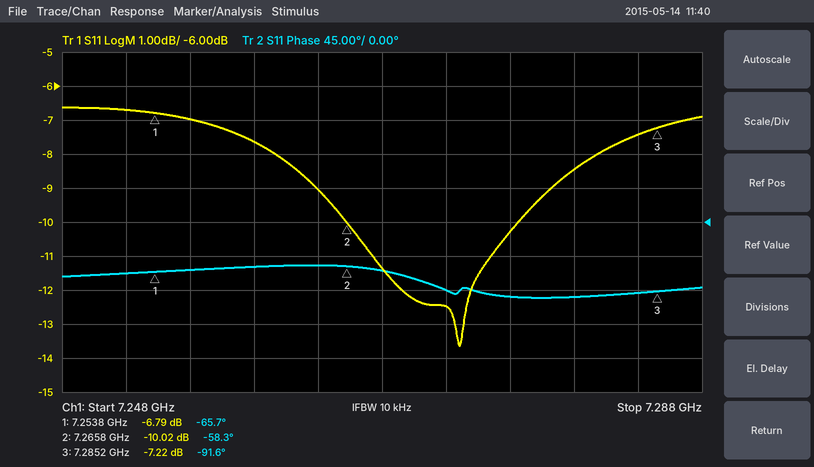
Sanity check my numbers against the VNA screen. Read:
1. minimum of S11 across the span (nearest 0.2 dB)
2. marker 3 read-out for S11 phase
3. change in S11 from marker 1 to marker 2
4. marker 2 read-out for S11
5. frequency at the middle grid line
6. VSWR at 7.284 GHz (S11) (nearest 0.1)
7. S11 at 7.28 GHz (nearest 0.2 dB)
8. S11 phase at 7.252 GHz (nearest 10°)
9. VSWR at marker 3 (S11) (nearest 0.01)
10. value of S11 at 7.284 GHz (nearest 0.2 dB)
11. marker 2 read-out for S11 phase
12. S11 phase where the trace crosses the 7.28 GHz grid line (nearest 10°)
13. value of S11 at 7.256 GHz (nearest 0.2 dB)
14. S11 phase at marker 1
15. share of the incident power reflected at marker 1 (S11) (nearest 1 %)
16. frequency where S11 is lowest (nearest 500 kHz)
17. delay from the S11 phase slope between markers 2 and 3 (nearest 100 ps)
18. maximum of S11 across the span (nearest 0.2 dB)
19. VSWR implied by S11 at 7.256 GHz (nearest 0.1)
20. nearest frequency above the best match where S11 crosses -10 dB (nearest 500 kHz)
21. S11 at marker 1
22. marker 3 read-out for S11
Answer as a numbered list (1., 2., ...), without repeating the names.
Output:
1. -13.6 dB
2. -91.6°
3. -3.23 dB
4. -10.02 dB
5. 7.268 GHz
6. 2.5
7. -8.4 dB
8. -70°
9. 2.54
10. -7.4 dB
11. -58.3°
12. -100°
13. -7.0 dB
14. -65.7°
15. 21 %
16. 7.2730 GHz
17. 4.8 ns
18. -6.6 dB
19. 2.6
20. 7.2765 GHz
21. -6.79 dB
22. -7.22 dB
